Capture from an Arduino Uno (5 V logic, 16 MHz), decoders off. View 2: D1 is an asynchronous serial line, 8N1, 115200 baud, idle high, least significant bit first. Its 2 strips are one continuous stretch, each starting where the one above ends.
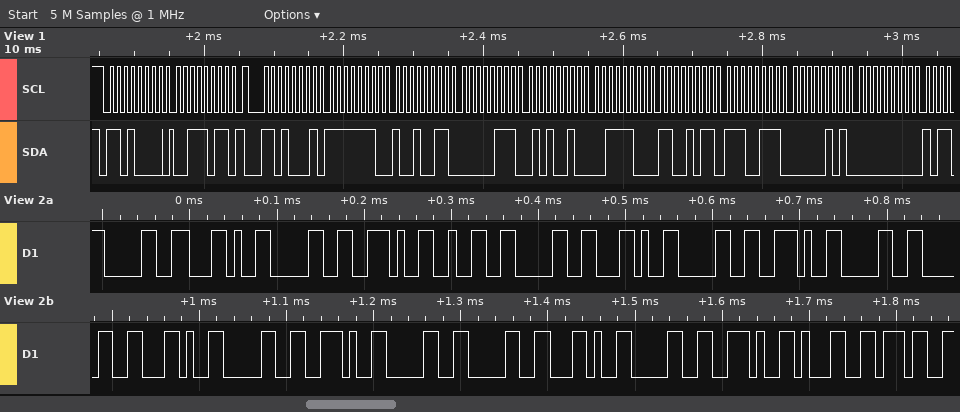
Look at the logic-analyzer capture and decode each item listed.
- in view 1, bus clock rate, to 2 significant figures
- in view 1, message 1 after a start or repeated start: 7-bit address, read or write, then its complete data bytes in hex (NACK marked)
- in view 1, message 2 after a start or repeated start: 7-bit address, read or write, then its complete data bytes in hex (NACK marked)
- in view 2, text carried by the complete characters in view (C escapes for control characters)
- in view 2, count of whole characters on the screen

100 kHz
0x68 write: 3B
0x68 read: FE 93 07 52 3C CB E7 05 00
"0,0.20,0.00,0.00,0.17"
21
